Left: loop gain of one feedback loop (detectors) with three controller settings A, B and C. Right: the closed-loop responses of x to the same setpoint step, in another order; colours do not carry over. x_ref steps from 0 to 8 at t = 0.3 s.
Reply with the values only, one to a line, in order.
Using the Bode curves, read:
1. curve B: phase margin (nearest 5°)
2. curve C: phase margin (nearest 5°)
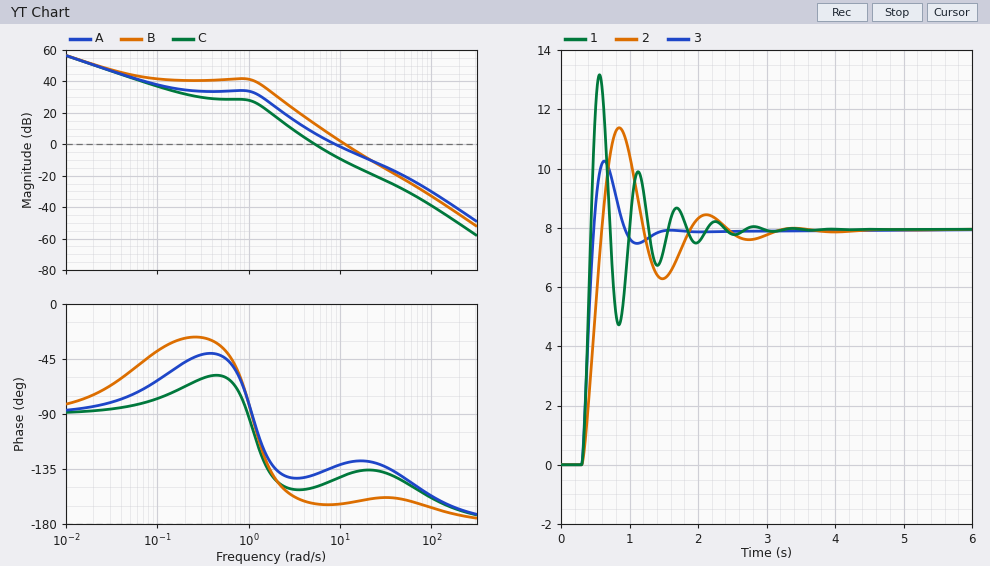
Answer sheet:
15°
30°
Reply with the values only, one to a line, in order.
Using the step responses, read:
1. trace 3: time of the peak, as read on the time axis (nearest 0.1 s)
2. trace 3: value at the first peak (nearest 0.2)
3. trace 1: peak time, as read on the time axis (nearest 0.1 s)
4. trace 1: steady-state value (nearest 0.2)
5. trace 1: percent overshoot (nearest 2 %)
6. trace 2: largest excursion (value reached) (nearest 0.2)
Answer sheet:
0.6 s
10.2
0.6 s
8.0
64 %
11.4
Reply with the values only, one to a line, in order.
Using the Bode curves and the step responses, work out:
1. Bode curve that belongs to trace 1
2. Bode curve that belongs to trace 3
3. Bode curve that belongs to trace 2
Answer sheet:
B
A
C
